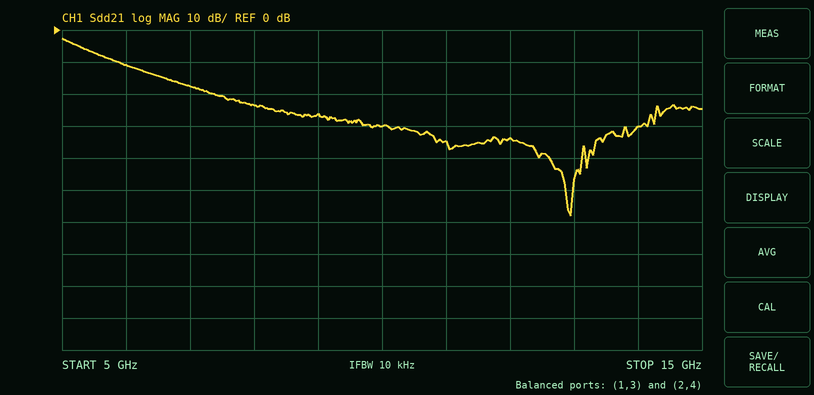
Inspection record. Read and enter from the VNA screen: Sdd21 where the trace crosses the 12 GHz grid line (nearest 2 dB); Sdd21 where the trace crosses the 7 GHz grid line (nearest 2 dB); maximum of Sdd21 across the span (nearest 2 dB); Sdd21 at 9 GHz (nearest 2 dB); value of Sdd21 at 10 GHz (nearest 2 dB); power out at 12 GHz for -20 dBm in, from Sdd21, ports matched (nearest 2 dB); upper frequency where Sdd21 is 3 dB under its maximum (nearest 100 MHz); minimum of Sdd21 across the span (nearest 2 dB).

-34 dB
-18 dB
-2 dB
-26 dB
-30 dB
-54 dBm
5.3 GHz
-58 dB
